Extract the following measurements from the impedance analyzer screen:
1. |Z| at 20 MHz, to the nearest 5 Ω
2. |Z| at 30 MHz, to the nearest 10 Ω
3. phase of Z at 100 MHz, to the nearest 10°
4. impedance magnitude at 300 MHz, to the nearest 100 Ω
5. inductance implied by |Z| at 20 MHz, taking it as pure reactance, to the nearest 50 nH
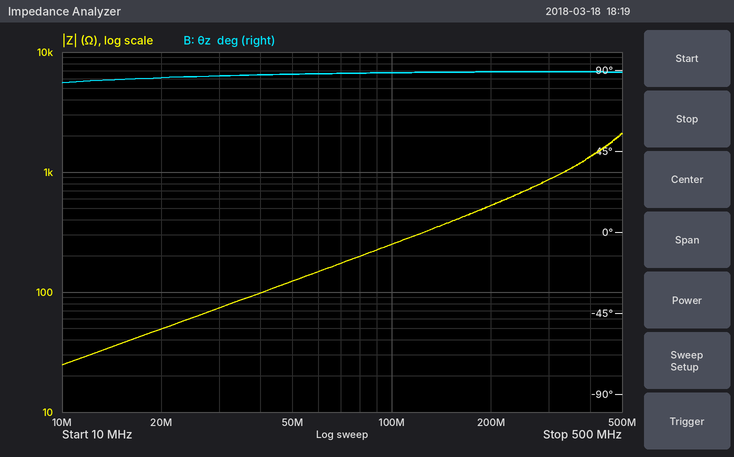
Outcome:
50 Ω
70 Ω
90°
900 Ω
400 nH
